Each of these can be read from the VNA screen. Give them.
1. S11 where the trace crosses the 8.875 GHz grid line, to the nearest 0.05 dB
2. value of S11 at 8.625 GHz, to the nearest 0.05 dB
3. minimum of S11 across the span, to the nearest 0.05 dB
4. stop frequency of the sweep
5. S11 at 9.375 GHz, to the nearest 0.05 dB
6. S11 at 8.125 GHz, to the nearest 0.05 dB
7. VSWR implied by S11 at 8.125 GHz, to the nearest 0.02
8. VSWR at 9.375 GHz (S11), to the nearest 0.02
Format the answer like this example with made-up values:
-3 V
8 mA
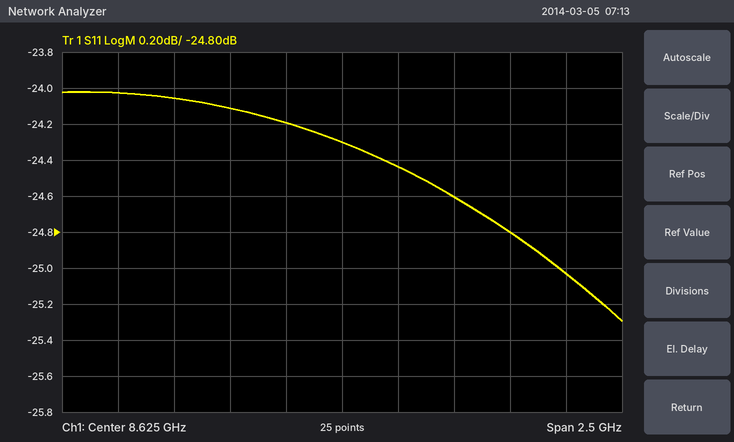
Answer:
-24.45 dB
-24.30 dB
-25.30 dB
9.875 GHz
-24.80 dB
-24.10 dB
1.14
1.12
